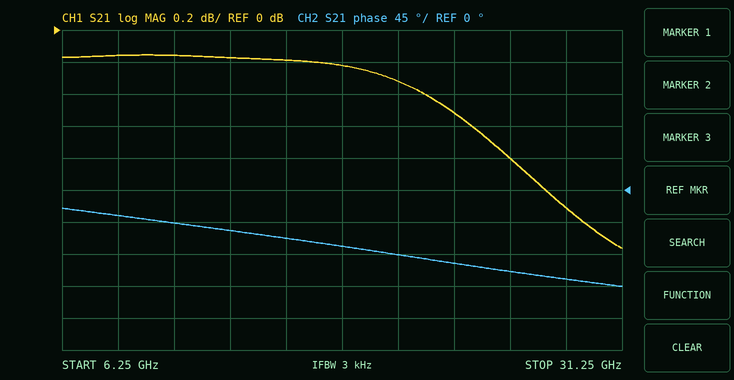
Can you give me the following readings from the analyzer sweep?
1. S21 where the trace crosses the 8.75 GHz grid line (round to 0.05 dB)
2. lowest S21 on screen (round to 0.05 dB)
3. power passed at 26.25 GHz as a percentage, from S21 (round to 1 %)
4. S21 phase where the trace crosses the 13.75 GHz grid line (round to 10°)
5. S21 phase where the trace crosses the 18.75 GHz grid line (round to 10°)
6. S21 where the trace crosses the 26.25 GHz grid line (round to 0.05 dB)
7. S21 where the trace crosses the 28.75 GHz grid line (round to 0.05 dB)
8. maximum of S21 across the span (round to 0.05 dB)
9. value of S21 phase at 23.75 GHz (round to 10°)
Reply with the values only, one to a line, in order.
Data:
-0.15 dB
-1.35 dB
83 %
-60°
-80°
-0.80 dB
-1.10 dB
-0.15 dB
-100°
